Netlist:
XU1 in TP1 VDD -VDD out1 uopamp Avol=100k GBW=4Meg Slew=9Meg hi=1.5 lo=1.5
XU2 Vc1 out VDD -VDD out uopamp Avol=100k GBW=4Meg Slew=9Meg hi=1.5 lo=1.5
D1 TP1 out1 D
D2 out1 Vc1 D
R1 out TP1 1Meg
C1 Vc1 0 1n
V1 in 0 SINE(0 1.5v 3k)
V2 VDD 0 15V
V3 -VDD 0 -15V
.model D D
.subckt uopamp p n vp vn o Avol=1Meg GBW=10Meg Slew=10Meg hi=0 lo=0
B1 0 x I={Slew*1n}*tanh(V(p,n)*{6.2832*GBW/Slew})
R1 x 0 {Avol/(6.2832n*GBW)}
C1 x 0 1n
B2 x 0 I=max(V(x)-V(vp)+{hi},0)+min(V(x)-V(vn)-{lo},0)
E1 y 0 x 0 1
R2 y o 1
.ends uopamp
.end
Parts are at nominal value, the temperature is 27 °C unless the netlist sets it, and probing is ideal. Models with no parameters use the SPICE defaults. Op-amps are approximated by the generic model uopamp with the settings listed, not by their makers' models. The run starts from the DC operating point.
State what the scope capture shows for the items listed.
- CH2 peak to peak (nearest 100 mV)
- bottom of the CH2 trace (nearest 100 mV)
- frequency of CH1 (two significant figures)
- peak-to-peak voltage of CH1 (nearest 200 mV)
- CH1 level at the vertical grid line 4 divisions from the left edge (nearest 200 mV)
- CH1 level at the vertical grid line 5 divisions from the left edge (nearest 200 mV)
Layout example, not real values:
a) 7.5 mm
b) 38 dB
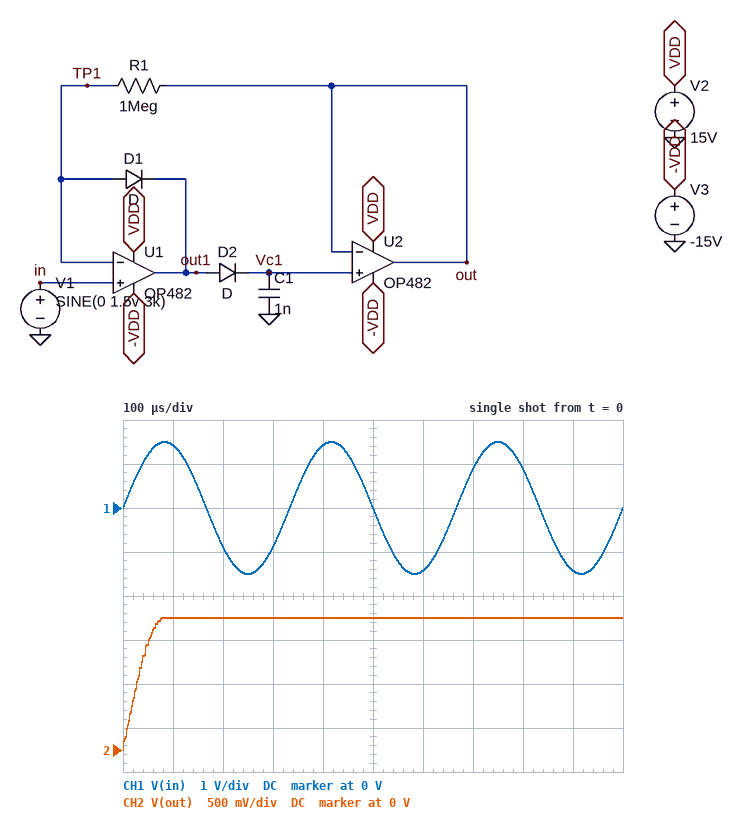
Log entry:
a) 1.5 V
b) 0 V
c) 3.0 kHz
d) 3.0 V
e) 1.4 V
f) 0 V
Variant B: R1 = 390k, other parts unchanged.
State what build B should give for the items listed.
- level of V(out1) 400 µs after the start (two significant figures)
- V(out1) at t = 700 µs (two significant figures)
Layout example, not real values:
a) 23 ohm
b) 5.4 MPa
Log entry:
a) 990 mV
b) 390 mV
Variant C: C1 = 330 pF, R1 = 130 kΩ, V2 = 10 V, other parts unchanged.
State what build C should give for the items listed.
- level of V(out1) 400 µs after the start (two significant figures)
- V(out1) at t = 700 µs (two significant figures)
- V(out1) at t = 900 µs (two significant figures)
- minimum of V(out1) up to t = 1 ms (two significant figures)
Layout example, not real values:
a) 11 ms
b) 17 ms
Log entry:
a) 960 mV
b) 360 mV
c) -2.0 V
d) -2.1 V
